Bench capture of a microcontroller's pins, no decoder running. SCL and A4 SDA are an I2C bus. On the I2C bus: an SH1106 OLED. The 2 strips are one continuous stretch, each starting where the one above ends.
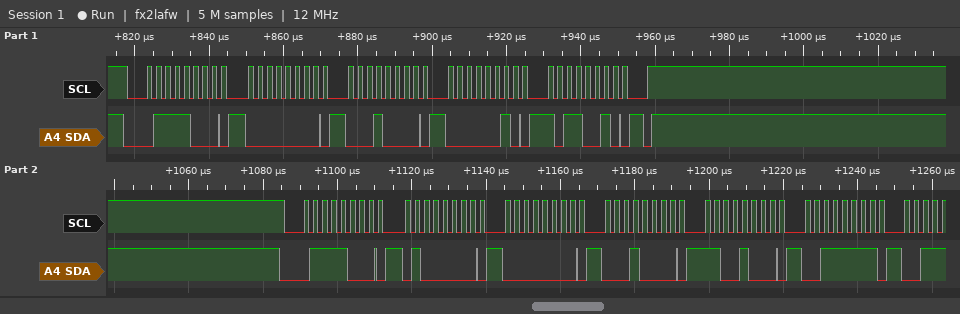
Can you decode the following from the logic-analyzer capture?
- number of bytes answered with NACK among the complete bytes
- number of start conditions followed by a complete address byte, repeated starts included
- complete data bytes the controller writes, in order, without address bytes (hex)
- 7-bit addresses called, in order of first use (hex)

0
2
00 10 02 B2 40 00 10 C8 3F
0x3C
